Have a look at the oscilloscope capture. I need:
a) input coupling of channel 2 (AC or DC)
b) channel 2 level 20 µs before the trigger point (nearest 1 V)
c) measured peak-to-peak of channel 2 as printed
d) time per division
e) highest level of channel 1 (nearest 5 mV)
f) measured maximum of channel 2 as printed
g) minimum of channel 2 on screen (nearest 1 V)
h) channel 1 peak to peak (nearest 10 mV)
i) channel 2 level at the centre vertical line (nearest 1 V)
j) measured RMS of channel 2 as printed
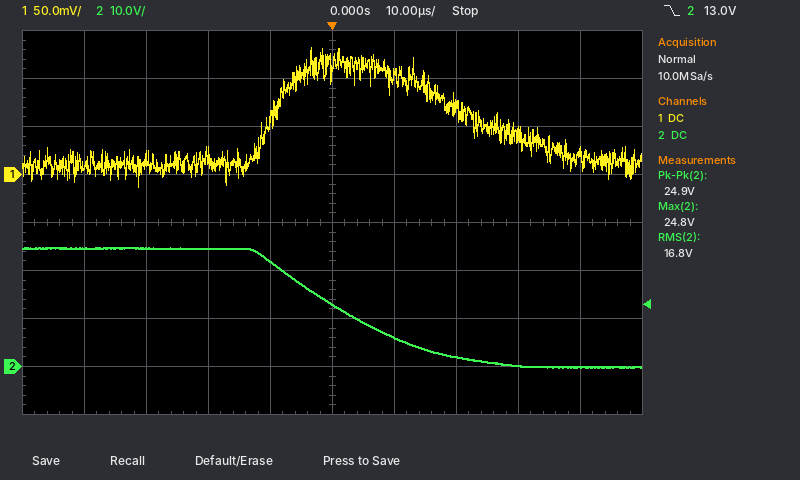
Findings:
DC
25 V
24.9 V
10 µs
130 mV
24.8 V
0 V
140 mV
13 V
16.8 V
